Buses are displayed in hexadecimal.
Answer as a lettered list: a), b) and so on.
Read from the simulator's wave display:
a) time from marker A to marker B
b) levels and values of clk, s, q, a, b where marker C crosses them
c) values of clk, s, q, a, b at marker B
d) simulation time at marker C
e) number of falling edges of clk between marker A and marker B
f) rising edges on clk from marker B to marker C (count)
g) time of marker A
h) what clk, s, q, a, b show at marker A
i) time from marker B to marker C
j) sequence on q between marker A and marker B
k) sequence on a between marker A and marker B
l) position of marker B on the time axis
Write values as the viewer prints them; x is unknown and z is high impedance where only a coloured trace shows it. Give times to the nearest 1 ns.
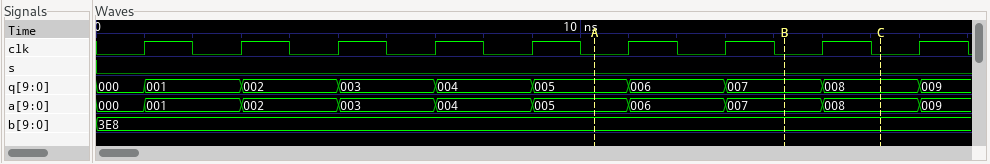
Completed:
a) 4 ns
b) clk=0, s=0, q=008, a=008, b=3E8
c) clk=0, s=0, q=007, a=007, b=3E8
d) 16 ns
e) 2
f) 1
g) 10 ns
h) clk=0, s=0, q=005, a=005, b=3E8
i) 2 ns
j) 005, 006, 007
k) 005, 006, 007
l) 14 ns
